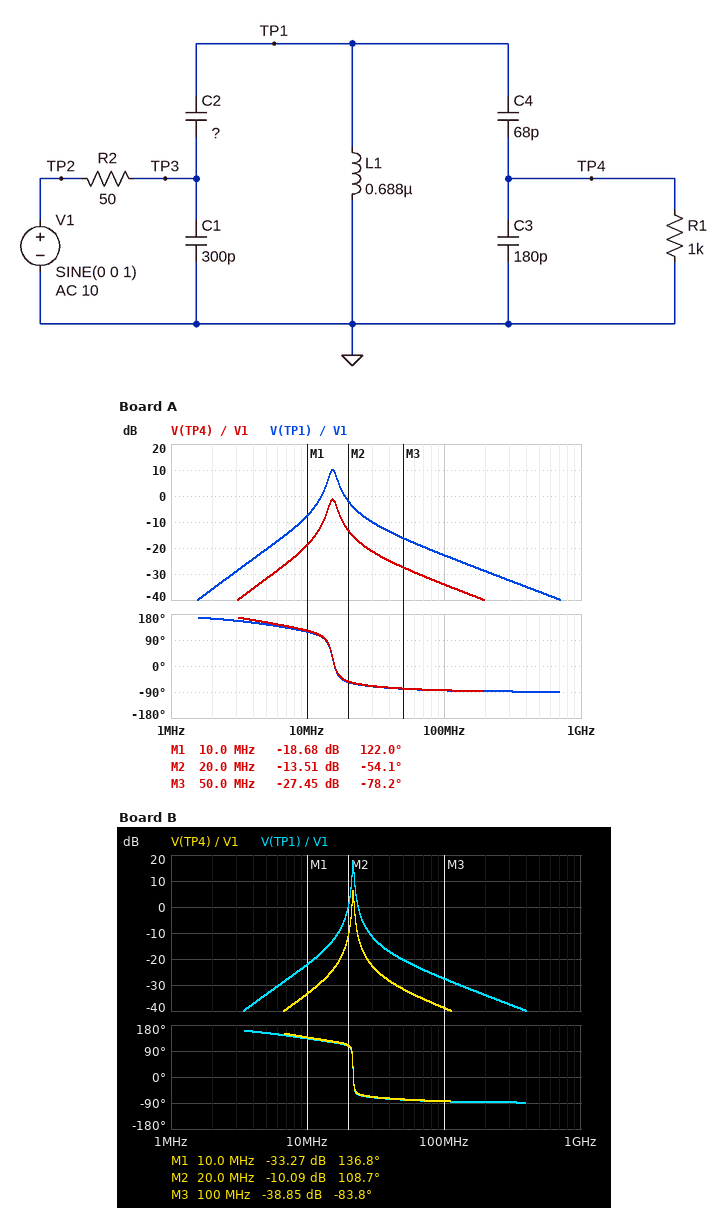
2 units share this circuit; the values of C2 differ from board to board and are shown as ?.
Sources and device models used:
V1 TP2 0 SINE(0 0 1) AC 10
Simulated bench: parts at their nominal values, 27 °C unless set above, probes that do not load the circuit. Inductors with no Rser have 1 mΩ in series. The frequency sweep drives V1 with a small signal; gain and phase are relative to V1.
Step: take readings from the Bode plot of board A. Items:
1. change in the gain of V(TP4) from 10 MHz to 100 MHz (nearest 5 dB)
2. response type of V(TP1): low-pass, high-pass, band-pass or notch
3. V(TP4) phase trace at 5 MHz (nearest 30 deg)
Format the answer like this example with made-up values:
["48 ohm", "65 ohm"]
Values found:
["-15 dB", "band-pass", "150 deg"]
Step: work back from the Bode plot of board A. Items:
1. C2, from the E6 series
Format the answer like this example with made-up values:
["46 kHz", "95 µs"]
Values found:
["150 pF"]
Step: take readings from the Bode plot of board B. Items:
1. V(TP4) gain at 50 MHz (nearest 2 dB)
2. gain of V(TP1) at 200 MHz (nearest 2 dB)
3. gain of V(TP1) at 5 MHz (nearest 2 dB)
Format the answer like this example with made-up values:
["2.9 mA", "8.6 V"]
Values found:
["-32 dB", "-34 dB", "-34 dB"]
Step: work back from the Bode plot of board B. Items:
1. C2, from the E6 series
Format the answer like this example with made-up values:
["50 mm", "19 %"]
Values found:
["33 pF"]
